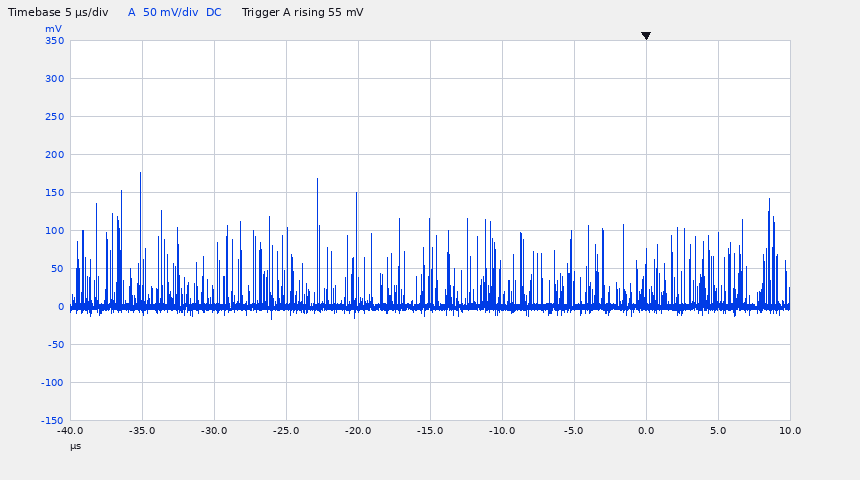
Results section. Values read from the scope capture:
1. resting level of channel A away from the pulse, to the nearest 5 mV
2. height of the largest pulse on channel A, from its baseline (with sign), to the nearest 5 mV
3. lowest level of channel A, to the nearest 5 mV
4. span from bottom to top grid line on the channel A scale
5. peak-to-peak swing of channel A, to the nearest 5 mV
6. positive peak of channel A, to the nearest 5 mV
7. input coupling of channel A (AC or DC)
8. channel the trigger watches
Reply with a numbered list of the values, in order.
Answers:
1. 0 mV
2. +175 mV
3. -15 mV
4. 500 mV
5. 190 mV
6. 175 mV
7. DC
8. channel A
